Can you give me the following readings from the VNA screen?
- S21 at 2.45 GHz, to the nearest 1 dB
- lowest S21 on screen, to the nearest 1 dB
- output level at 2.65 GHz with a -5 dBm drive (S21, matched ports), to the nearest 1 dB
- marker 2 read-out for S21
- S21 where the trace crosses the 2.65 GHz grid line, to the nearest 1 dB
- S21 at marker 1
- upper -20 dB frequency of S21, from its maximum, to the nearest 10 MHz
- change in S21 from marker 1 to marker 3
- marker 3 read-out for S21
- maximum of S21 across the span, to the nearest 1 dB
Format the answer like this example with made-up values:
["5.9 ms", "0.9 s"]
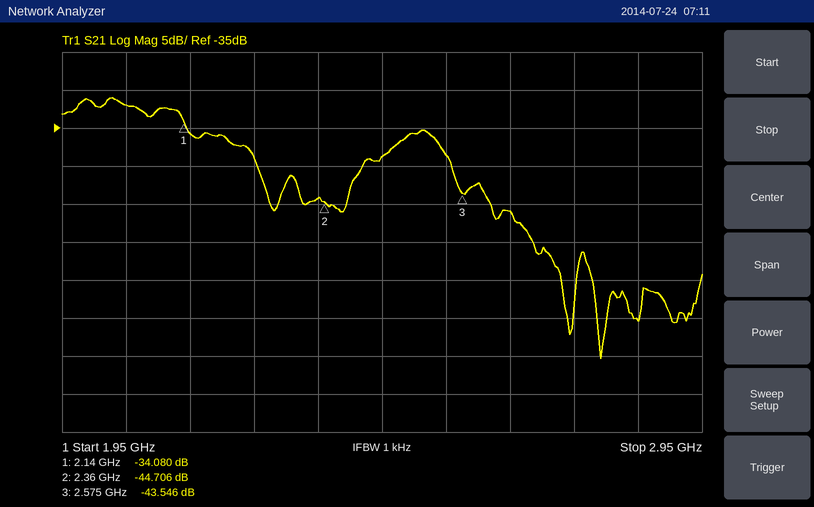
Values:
["-39 dB", "-65 dB", "-51 dBm", "-44.706 dB", "-46 dB", "-34.080 dB", "2.69 GHz", "-9.466 dB", "-43.546 dB", "-31 dB"]
